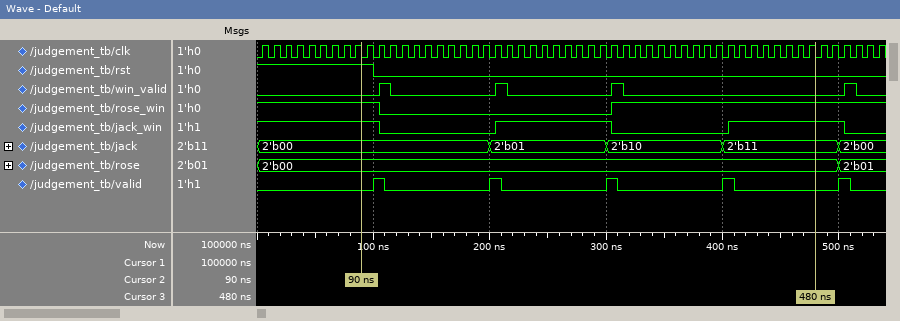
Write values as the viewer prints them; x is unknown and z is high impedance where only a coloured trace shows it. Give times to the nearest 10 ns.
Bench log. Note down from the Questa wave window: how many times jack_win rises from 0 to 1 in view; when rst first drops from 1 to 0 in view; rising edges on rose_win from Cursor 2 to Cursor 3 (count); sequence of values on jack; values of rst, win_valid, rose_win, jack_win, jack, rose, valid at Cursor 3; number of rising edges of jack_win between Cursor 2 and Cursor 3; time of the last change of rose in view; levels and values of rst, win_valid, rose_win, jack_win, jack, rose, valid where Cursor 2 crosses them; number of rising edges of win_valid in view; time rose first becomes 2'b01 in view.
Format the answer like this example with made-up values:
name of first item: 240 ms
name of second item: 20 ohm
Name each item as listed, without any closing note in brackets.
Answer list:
how many times jack_win rises from 0 to 1 in view: 2
when rst first drops from 1 to 0 in view: 100 ns
rising edges on rose_win from Cursor 2 to Cursor 3: 1
sequence of values on jack: 2'b00, 2'b01, 2'b10, 2'b11, 2'b00
values of rst, win_valid, rose_win, jack_win, jack, rose, valid at Cursor 3: rst=0, win_valid=0, rose_win=1, jack_win=1, jack=2'b11, rose=2'b00, valid=0
number of rising edges of jack_win between Cursor 2 and Cursor 3: 2
time of the last change of rose in view: 500 ns
levels and values of rst, win_valid, rose_win, jack_win, jack, rose, valid where Cursor 2 crosses them: rst=1, win_valid=0, rose_win=1, jack_win=1, jack=2'b00, rose=2'b00, valid=0
number of rising edges of win_valid in view: 4
time rose first becomes 2'b01 in view: 500 ns
